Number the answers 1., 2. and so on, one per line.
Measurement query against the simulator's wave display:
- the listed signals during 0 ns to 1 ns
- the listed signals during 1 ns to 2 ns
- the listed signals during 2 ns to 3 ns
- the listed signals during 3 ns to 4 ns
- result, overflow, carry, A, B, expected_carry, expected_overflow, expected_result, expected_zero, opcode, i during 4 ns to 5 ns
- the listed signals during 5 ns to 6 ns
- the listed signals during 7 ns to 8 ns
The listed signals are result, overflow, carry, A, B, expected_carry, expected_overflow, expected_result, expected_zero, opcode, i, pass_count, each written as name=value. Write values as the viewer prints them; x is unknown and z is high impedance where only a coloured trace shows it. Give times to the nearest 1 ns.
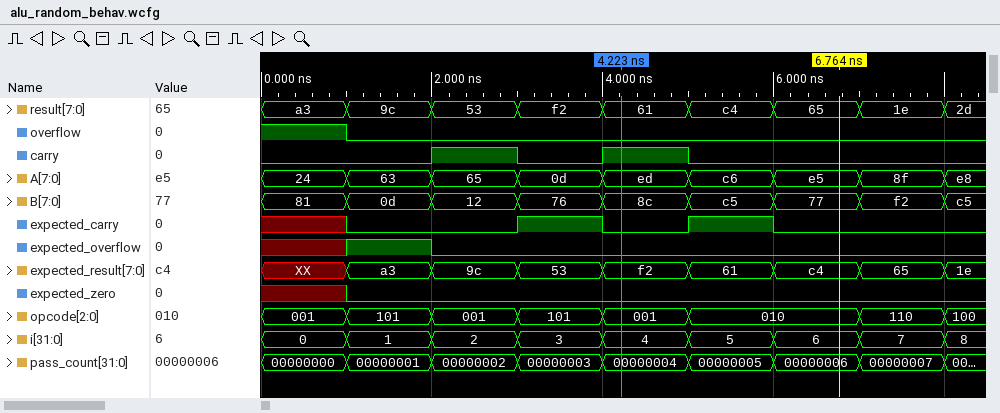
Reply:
1. result=a3, overflow=1, carry=0, A=24, B=81, expected_carry=x, expected_overflow=x, expected_result=XX, expected_zero=x, opcode=001, i=0, pass_count=00000000
2. result=9c, overflow=0, carry=0, A=63, B=0d, expected_carry=0, expected_overflow=1, expected_result=a3, expected_zero=0, opcode=101, i=1, pass_count=00000001
3. result=53, overflow=0, carry=1, A=65, B=12, expected_carry=0, expected_overflow=0, expected_result=9c, expected_zero=0, opcode=001, i=2, pass_count=00000002
4. result=f2, overflow=0, carry=0, A=0d, B=76, expected_carry=1, expected_overflow=0, expected_result=53, expected_zero=0, opcode=101, i=3, pass_count=00000003
5. result=61, overflow=0, carry=1, A=ed, B=8c, expected_carry=0, expected_overflow=0, expected_result=f2, expected_zero=0, opcode=001, i=4
6. result=c4, overflow=0, carry=0, A=c6, B=c5, expected_carry=1, expected_overflow=0, expected_result=61, expected_zero=0, opcode=010, i=5, pass_count=00000005
7. result=1e, overflow=0, carry=0, A=8f, B=f2, expected_carry=0, expected_overflow=0, expected_result=65, expected_zero=0, opcode=110, i=7, pass_count=00000007
